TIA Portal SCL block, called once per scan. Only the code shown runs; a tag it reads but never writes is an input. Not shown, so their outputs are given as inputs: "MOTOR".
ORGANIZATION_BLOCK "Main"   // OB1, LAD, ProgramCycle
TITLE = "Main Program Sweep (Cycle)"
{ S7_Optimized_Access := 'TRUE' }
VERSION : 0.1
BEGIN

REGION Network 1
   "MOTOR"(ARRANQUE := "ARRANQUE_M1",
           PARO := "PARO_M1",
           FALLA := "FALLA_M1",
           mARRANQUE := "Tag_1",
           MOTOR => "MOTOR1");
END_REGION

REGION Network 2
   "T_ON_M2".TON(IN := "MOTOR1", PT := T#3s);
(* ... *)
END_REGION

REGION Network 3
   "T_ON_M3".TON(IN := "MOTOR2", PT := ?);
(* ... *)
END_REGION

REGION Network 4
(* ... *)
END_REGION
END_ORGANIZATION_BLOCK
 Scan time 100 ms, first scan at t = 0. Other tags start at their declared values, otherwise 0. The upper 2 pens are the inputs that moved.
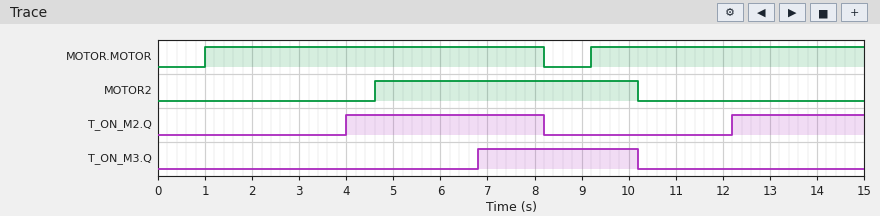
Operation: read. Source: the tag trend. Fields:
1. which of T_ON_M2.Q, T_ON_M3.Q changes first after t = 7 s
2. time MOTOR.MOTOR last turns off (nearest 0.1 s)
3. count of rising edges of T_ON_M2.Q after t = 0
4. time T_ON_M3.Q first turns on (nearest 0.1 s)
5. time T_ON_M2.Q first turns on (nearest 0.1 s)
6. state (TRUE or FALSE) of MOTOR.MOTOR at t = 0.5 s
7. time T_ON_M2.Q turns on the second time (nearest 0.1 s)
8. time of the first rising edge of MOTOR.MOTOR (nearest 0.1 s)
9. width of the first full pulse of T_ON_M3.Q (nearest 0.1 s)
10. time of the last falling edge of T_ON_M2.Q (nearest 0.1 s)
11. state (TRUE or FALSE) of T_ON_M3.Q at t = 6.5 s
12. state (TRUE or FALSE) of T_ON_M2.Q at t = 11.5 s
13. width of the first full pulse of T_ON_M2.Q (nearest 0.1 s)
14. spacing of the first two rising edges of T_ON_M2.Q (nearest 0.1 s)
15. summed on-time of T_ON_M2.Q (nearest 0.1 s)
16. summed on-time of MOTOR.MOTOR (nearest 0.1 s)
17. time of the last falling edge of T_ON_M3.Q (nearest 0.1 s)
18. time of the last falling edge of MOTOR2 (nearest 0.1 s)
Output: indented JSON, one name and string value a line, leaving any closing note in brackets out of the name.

{
  "which of T_ON_M2.Q, T_ON_M3.Q changes first after t = 7 s": "T_ON_M2.Q",
  "time MOTOR.MOTOR last turns off": "8.2 s",
  "count of rising edges of T_ON_M2.Q after t = 0": "2",
  "time T_ON_M3.Q first turns on": "6.8 s",
  "time T_ON_M2.Q first turns on": "4.0 s",
  "state (TRUE or FALSE) of MOTOR.MOTOR at t = 0.5 s": "FALSE",
  "time T_ON_M2.Q turns on the second time": "12.2 s",
  "time of the first rising edge of MOTOR.MOTOR": "1.0 s",
  "width of the first full pulse of T_ON_M3.Q": "3.4 s",
  "time of the last falling edge of T_ON_M2.Q": "8.2 s",
  "state (TRUE or FALSE) of T_ON_M3.Q at t = 6.5 s": "FALSE",
  "state (TRUE or FALSE) of T_ON_M2.Q at t = 11.5 s": "FALSE",
  "width of the first full pulse of T_ON_M2.Q": "4.2 s",
  "spacing of the first two rising edges of T_ON_M2.Q": "8.2 s",
  "summed on-time of T_ON_M2.Q": "7.0 s",
  "summed on-time of MOTOR.MOTOR": "13.0 s",
  "time of the last falling edge of T_ON_M3.Q": "10.2 s",
  "time of the last falling edge of MOTOR2": "10.2 s"
}
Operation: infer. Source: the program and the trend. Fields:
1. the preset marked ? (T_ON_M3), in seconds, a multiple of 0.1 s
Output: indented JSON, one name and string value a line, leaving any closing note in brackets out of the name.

{
  "the preset marked ? (T_ON_M3), in seconds, a multiple of 0.1 s": "2.2 s"
}
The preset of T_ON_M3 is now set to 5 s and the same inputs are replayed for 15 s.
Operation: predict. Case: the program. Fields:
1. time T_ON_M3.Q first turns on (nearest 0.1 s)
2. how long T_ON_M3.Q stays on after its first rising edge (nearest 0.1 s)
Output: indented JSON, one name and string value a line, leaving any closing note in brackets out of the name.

{
  "time T_ON_M3.Q first turns on": "9.6 s",
  "how long T_ON_M3.Q stays on after its first rising edge": "0.6 s"
}
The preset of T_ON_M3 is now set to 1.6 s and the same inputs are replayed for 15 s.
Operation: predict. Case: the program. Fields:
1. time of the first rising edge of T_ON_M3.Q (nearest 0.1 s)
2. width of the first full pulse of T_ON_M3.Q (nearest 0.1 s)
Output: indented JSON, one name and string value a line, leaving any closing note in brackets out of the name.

{
  "time of the first rising edge of T_ON_M3.Q": "6.2 s",
  "width of the first full pulse of T_ON_M3.Q": "4.0 s"
}
